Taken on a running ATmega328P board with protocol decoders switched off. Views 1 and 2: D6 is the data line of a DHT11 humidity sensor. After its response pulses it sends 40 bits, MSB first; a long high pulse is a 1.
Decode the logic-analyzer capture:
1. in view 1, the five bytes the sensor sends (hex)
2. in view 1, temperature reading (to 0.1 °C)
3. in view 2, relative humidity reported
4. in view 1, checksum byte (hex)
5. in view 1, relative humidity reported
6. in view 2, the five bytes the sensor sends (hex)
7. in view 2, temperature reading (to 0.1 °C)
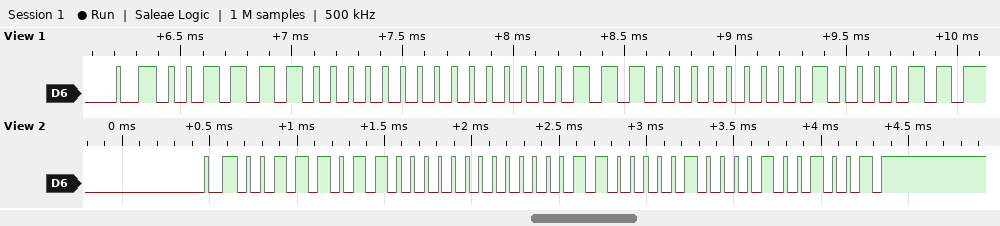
3C 00 07 00 43
7.0 °C
59 %
0x43
60 %
3B 00 06 08 49
6.8 °C
